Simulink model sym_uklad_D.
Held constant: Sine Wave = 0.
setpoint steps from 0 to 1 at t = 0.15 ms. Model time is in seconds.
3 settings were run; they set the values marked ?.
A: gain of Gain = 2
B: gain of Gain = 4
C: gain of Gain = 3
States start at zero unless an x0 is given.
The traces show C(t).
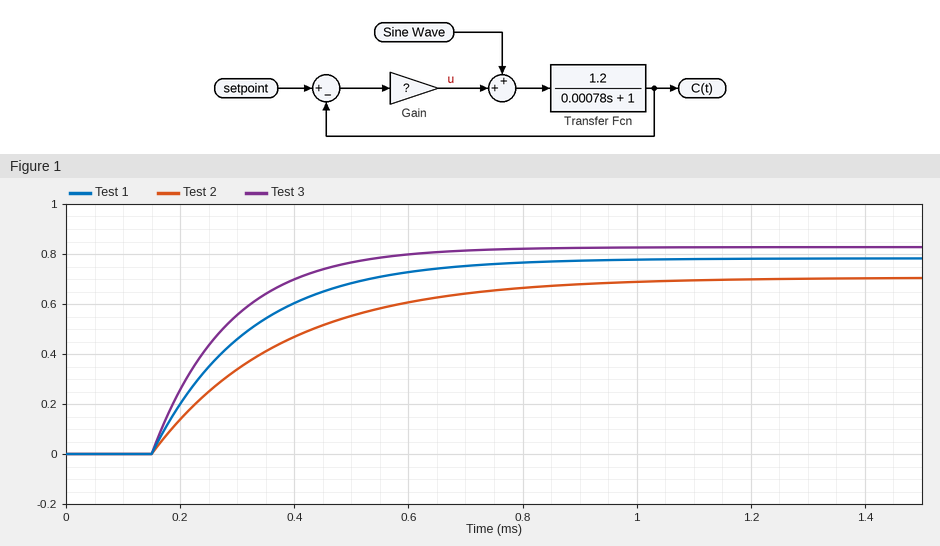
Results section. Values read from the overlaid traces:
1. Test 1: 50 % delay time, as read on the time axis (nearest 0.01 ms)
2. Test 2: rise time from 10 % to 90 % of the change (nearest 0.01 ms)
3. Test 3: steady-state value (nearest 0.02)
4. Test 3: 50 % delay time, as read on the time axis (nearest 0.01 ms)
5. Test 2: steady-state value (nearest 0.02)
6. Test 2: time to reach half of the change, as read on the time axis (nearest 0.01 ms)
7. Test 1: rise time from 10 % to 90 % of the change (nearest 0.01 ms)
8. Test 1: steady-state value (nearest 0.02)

0.27 ms
0.50 ms
0.82
0.24 ms
0.70
0.31 ms
0.37 ms
0.78
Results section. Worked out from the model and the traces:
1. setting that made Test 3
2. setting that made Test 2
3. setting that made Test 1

B
A
C
